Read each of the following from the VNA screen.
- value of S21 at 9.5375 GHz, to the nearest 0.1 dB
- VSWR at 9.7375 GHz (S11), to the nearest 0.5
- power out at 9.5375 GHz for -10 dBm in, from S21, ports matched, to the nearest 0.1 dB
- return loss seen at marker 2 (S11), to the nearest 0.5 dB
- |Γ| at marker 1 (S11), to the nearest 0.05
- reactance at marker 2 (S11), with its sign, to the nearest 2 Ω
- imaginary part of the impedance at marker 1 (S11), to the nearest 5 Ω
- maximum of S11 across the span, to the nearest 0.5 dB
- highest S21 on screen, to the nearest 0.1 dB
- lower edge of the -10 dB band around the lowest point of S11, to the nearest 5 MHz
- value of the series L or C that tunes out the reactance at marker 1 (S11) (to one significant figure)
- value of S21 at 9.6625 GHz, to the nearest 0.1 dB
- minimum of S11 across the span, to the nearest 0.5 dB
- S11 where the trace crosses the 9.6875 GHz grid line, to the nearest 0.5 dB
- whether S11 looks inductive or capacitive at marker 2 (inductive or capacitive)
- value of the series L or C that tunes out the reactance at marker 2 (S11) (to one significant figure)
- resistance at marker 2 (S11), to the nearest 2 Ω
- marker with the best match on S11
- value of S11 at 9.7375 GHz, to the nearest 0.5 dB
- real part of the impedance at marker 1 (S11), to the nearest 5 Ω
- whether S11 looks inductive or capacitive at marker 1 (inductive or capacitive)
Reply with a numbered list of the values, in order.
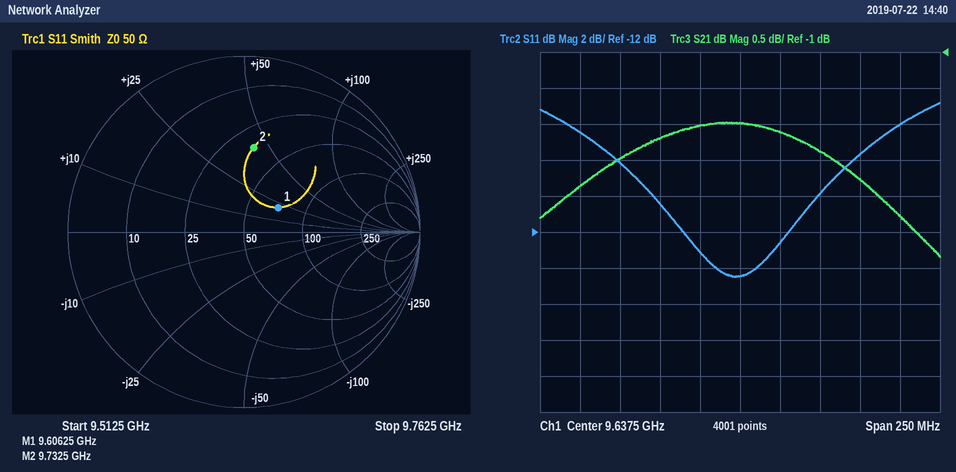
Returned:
1. -2.9 dB
2. 3.0
3. -12.9 dBm
4. 6.5 dB
5. 0.25
6. +42 Ω
7. +20 Ω
8. -5.0 dB
9. -2.0 dB
10. 9.585 GHz
11. 800 fF
12. -2.1 dB
13. -14.5 dB
14. -10.0 dB
15. inductive
16. 400 fF
17. 34 Ω
18. marker 1
19. -6.0 dB
20. 70 Ω
21. inductive
